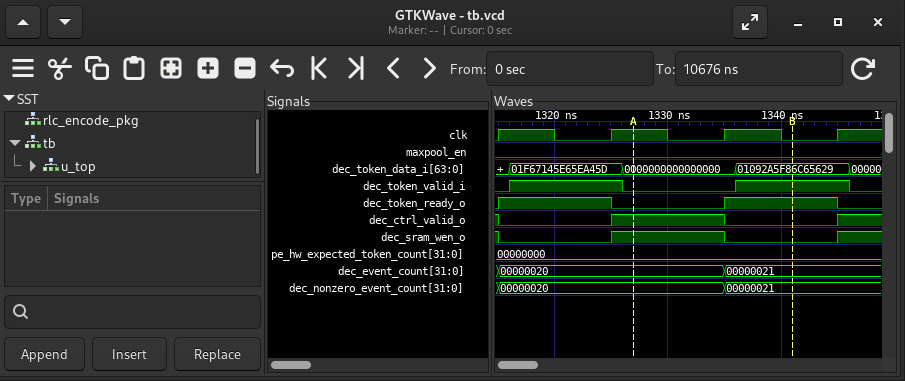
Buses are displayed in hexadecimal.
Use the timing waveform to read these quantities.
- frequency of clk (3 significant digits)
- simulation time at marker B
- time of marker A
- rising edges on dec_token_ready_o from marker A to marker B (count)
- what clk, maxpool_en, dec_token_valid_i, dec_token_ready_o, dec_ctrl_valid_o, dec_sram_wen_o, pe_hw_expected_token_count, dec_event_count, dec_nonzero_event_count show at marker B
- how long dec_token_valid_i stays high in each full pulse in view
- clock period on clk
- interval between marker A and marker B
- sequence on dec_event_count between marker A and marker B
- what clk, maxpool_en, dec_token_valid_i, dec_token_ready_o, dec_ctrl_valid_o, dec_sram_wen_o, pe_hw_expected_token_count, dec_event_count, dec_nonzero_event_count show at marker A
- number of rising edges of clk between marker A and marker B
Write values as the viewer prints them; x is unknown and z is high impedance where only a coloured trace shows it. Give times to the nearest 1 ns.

100 MHz
1341 ns
1327 ns
1
clk=0, maxpool_en=0, dec_token_valid_i=1, dec_token_ready_o=1, dec_ctrl_valid_o=0, dec_sram_wen_o=0, pe_hw_expected_token_count=00000000, dec_event_count=00000021, dec_nonzero_event_count=00000021
10 ns, 10 ns
10 ns
14 ns
00000020, 00000021
clk=1, maxpool_en=0, dec_token_valid_i=0, dec_token_ready_o=0, dec_ctrl_valid_o=1, dec_sram_wen_o=1, pe_hw_expected_token_count=00000000, dec_event_count=00000020, dec_nonzero_event_count=00000020
1
